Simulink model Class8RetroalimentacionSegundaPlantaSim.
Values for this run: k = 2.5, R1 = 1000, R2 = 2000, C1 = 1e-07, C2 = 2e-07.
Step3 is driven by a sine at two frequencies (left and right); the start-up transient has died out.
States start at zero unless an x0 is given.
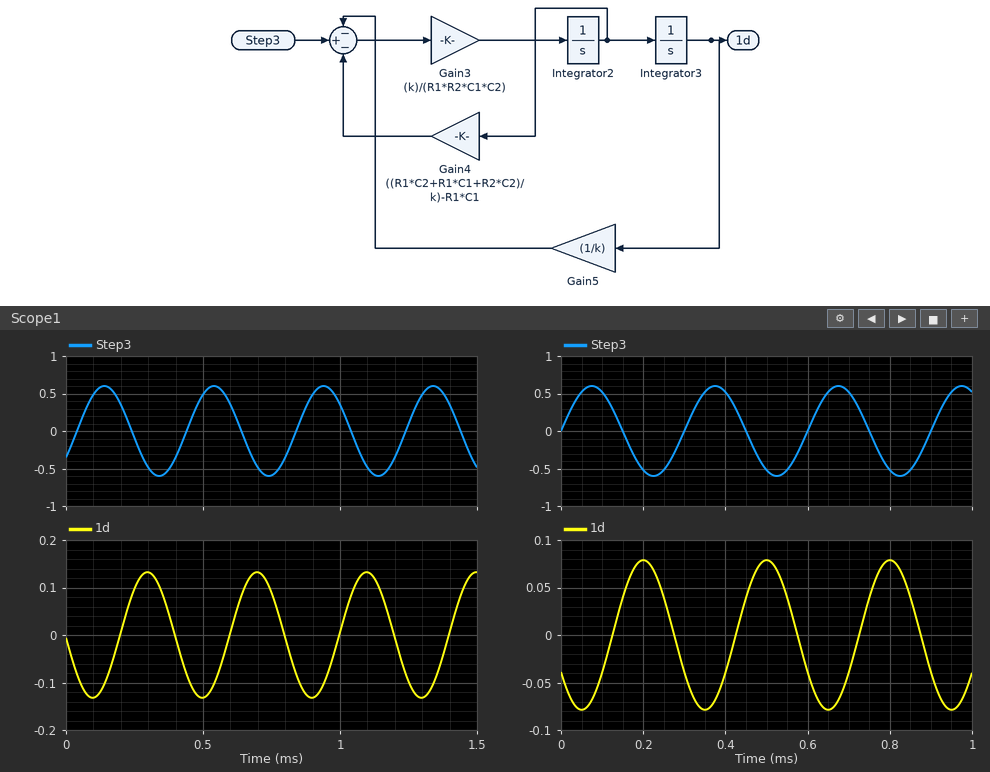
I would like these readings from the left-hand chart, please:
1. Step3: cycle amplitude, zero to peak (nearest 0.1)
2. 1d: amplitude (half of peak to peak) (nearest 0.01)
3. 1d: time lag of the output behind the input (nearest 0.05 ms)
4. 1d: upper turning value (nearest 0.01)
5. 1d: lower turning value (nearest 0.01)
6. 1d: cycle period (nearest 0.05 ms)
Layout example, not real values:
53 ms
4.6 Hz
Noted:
0.6
0.13
0.15 ms
0.13
-0.13
0.40 ms
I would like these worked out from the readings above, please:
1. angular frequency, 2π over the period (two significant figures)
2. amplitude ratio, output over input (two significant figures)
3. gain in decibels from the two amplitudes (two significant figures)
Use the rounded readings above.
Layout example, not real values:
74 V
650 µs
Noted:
16 rad/ms
0.22
-13 dB
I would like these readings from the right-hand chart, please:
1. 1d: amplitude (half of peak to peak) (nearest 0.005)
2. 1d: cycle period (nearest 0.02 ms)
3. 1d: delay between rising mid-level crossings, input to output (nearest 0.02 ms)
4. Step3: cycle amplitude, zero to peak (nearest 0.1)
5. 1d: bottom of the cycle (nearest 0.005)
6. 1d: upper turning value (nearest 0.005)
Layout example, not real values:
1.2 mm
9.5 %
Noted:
0.080
0.30 ms
0.12 ms
0.6
-0.080
0.080
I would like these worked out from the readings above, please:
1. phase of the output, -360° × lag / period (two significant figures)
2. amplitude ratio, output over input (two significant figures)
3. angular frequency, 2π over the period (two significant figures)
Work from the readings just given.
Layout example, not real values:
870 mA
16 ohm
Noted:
-140°
0.13
21 rad/ms
